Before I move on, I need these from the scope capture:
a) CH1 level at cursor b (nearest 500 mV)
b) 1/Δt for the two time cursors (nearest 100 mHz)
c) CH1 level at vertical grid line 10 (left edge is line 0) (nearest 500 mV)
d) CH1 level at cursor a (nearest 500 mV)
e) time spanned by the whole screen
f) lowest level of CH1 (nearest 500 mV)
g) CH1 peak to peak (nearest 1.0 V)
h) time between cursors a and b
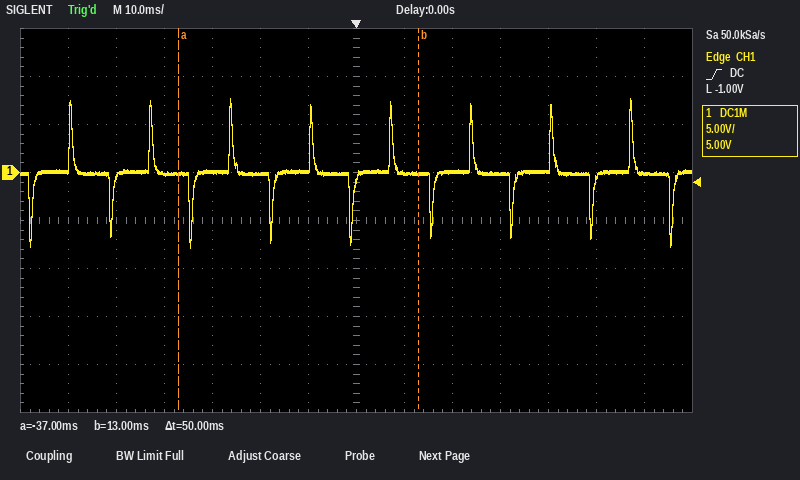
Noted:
0.0 V
20.0 Hz
0.0 V
0.0 V
140 ms
-8.0 V
16.0 V
50 ms
